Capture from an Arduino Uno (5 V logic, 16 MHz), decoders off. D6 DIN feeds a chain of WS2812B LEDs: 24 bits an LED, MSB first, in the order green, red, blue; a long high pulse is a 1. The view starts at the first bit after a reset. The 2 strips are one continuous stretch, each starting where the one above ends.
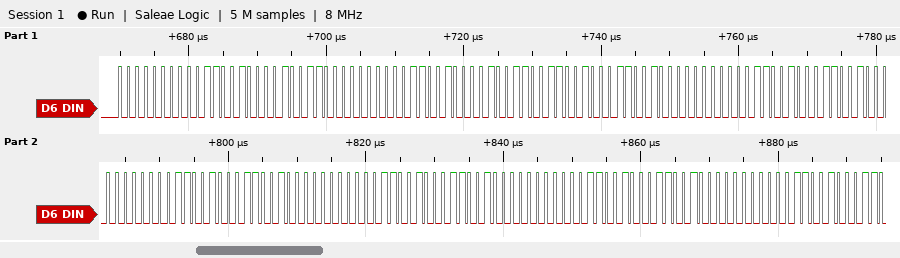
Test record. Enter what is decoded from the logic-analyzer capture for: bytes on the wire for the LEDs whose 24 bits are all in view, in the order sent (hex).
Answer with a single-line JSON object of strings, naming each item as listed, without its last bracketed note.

{"bytes on the wire for the LEDs whose 24 bits are all in view, in the order sent": "00 32 13 00 32 13 32 32 00 32 32 00 32 32 00 32 32 00 32 32 00"}
